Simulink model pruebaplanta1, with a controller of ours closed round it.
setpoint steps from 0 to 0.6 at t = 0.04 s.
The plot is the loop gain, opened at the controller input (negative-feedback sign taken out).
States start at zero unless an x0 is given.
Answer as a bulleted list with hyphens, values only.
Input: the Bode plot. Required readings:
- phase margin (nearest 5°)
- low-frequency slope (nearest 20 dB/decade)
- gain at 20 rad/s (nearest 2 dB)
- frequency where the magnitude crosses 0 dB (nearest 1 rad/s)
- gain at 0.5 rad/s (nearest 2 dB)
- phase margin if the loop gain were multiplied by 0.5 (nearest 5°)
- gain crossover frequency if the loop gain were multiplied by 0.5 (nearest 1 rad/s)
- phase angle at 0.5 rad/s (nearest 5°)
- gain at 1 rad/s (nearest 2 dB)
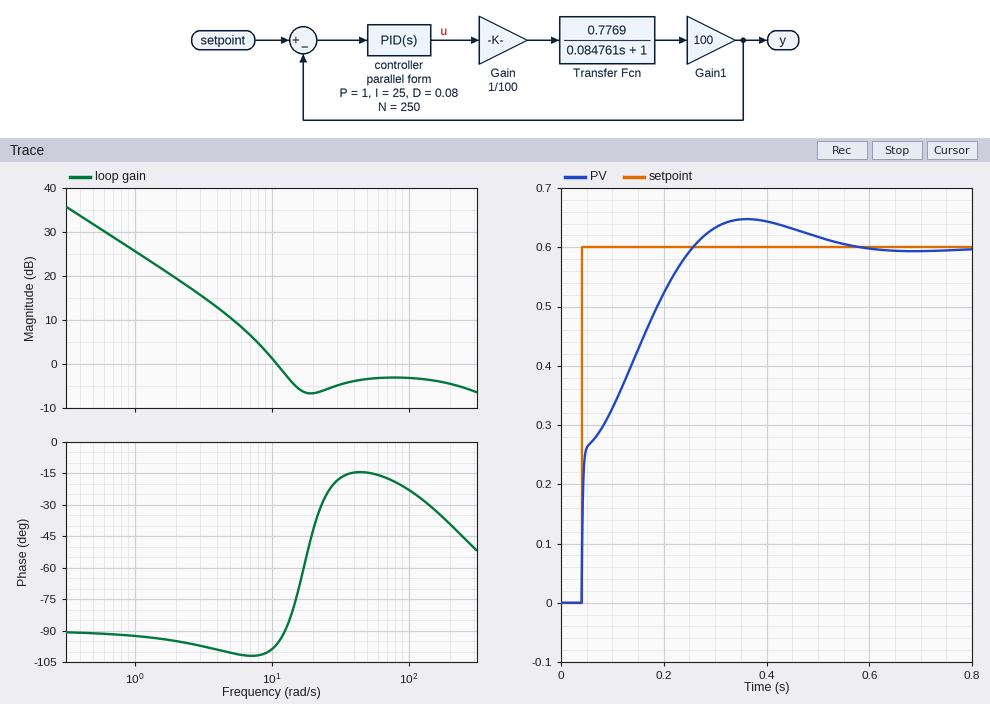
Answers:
- 85°
- -20 dB/decade
- -6 dB
- 11 rad/s
- 32 dB
- 80°
- 7 rad/s
- -90°
- 26 dB
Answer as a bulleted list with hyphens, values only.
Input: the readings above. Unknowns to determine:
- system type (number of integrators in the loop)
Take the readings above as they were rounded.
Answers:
- 1
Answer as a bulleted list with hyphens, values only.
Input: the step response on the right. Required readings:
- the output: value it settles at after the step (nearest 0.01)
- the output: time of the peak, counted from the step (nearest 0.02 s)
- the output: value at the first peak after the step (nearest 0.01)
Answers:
- 0.60
- 0.32 s
- 0.65
